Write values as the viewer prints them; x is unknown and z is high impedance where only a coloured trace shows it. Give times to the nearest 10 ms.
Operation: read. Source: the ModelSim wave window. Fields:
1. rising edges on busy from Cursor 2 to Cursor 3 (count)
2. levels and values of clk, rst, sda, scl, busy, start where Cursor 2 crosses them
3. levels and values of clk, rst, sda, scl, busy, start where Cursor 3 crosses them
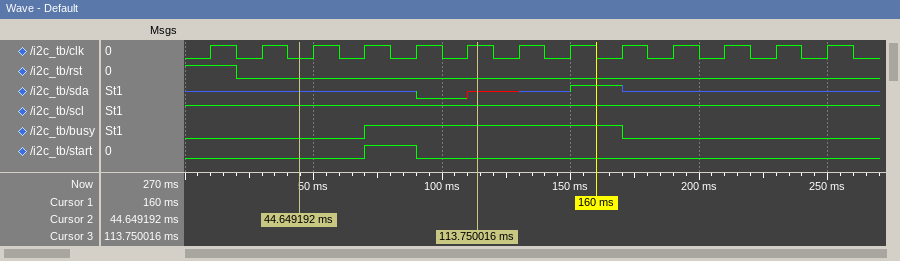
1
clk=0, rst=0, sda=z, scl=1, busy=0, start=0
clk=1, rst=0, sda=x, scl=1, busy=1, start=0
